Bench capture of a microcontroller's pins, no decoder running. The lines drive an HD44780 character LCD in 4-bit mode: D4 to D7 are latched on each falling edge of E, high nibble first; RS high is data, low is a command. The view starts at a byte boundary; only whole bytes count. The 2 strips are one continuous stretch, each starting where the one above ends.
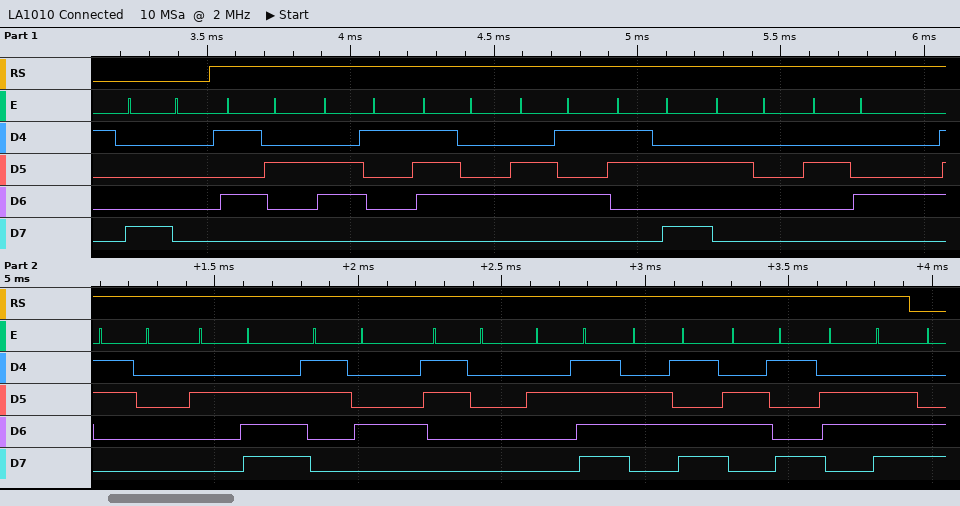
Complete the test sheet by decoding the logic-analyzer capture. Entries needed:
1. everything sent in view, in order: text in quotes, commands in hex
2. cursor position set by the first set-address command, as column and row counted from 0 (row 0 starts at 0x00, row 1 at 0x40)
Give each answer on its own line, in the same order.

0x80 "Rate: $0.40/min"
column 0, row 0
